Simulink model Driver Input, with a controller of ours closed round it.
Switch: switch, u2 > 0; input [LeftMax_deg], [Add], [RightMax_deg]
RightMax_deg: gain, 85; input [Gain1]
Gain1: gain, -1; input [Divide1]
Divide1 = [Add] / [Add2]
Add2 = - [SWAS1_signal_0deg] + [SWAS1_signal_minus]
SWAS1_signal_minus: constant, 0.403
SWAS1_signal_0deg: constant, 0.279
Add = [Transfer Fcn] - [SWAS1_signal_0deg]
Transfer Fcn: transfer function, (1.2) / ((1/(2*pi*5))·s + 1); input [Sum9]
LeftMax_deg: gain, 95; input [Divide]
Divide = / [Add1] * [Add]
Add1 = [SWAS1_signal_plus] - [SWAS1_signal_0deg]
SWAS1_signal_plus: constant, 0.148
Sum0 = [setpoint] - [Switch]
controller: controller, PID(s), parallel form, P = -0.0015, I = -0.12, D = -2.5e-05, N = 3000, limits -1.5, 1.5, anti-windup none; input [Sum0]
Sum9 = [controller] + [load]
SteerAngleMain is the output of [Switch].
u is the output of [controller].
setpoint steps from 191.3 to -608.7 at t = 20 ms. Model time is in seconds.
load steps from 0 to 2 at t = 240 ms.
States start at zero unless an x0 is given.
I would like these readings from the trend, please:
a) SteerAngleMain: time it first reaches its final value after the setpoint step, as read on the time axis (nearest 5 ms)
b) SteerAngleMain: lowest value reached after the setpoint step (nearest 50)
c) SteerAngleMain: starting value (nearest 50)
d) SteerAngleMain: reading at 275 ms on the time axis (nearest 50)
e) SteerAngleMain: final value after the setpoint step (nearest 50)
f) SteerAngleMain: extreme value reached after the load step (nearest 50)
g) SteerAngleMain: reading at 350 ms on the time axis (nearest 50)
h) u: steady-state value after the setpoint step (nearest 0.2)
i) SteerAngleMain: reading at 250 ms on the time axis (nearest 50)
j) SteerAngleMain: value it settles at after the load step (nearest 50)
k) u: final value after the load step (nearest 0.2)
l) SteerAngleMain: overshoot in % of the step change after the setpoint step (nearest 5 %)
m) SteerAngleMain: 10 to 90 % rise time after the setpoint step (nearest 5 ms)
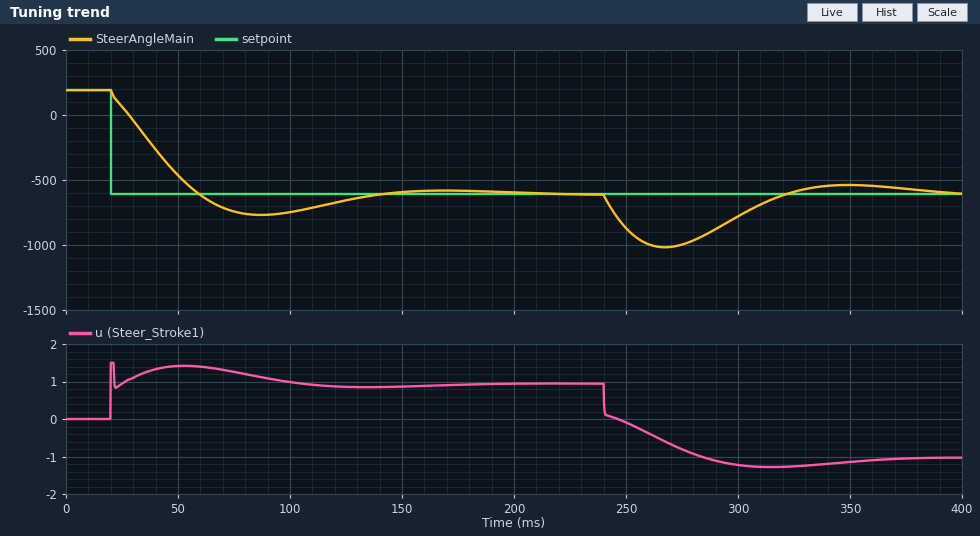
60 ms
-750
200
-1000
-600
-1000
-550
1.0
-850
-600
-1.0
20 %
30 ms
